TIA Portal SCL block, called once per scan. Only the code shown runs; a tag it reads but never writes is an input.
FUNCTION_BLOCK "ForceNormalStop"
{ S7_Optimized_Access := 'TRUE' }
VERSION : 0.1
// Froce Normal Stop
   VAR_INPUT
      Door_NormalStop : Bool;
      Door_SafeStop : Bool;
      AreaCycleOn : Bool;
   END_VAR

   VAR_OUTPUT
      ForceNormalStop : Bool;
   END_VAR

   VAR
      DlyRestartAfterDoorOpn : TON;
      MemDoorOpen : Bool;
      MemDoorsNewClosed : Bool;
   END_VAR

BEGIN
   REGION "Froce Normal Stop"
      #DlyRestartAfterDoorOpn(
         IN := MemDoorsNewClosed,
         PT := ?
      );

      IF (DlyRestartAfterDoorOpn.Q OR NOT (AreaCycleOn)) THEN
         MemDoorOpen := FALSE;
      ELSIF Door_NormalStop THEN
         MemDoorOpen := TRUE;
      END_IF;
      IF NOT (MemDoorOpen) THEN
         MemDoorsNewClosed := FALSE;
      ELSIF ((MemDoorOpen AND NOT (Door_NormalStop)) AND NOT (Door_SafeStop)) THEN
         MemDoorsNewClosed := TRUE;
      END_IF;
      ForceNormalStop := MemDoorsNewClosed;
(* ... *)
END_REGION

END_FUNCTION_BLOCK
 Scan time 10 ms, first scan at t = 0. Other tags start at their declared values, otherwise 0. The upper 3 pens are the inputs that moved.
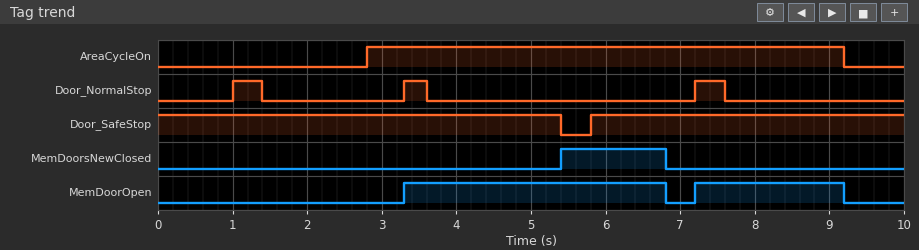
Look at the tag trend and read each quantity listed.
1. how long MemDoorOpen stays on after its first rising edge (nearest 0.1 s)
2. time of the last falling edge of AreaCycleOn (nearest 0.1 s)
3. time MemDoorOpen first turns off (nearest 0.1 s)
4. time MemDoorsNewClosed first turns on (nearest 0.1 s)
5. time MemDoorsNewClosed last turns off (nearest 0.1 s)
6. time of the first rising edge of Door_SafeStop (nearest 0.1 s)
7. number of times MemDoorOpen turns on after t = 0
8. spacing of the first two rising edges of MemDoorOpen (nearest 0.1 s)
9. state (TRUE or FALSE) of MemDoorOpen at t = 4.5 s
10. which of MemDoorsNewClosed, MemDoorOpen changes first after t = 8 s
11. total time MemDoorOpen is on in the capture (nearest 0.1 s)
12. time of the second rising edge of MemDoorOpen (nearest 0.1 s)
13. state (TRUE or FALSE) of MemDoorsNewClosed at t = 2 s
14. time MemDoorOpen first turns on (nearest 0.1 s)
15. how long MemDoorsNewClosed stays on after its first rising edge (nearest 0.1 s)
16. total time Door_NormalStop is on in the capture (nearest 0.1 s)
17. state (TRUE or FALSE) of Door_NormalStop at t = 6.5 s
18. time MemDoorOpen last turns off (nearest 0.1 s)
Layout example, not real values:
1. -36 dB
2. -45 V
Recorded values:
1. 3.5 s
2. 9.2 s
3. 6.8 s
4. 5.4 s
5. 6.8 s
6. 5.8 s
7. 2
8. 3.9 s
9. TRUE
10. MemDoorOpen
11. 5.5 s
12. 7.2 s
13. FALSE
14. 3.3 s
15. 1.4 s
16. 1.1 s
17. FALSE
18. 9.2 s
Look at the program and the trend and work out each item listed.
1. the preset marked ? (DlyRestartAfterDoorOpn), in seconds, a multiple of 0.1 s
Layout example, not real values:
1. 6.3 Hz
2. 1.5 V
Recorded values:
1. 1.4 s
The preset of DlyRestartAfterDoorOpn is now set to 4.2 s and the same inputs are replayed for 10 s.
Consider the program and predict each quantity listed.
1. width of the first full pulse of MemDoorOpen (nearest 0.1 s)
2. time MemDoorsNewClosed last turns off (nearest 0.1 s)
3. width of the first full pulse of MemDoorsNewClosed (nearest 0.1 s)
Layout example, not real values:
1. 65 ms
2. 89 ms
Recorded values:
1. 5.9 s
2. 9.2 s
3. 3.8 s
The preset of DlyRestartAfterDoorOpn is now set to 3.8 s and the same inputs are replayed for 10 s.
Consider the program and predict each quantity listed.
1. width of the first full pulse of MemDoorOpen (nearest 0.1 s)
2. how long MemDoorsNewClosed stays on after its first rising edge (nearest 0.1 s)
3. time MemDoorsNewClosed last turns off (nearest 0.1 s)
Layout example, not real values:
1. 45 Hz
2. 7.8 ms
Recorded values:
1. 5.9 s
2. 3.8 s
3. 9.2 s
